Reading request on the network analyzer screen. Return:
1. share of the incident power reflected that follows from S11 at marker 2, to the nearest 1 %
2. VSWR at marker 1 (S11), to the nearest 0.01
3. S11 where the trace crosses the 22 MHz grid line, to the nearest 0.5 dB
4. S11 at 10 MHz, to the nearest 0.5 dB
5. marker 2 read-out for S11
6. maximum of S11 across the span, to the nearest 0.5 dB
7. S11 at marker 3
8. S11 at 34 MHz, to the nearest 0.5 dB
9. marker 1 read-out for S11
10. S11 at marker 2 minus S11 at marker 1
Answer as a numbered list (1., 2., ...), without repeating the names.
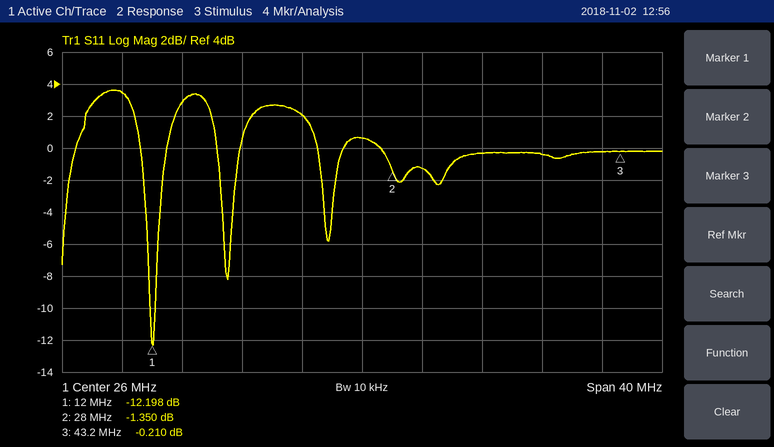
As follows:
1. 73 %
2. 1.65
3. 2.0 dB
4. 3.5 dB
5. -1.350 dB
6. 3.5 dB
7. -0.210 dB
8. -0.5 dB
9. -12.198 dB
10. 10.848 dB
